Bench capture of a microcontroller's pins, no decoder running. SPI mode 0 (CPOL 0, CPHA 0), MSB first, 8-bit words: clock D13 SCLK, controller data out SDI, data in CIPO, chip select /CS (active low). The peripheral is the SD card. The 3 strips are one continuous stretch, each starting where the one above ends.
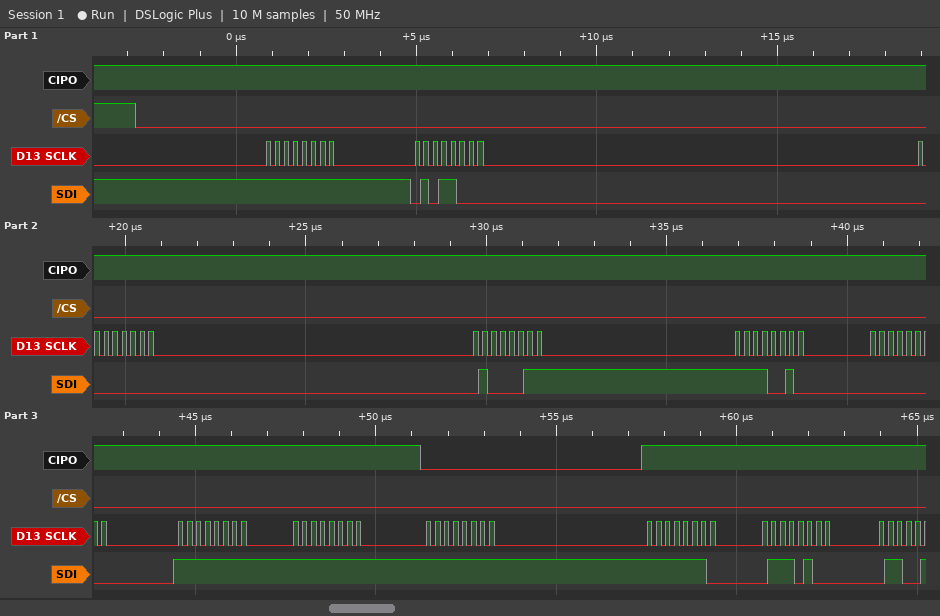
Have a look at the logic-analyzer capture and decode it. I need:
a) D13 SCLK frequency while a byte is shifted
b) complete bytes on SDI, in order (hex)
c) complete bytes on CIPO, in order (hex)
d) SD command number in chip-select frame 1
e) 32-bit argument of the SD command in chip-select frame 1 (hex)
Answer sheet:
4 MHz
FF 58 00 43 F2 00 FF FF FF FE 74
FF FF FF FF FF FF FF FF 00 FF FF
CMD24
0x0043F200
